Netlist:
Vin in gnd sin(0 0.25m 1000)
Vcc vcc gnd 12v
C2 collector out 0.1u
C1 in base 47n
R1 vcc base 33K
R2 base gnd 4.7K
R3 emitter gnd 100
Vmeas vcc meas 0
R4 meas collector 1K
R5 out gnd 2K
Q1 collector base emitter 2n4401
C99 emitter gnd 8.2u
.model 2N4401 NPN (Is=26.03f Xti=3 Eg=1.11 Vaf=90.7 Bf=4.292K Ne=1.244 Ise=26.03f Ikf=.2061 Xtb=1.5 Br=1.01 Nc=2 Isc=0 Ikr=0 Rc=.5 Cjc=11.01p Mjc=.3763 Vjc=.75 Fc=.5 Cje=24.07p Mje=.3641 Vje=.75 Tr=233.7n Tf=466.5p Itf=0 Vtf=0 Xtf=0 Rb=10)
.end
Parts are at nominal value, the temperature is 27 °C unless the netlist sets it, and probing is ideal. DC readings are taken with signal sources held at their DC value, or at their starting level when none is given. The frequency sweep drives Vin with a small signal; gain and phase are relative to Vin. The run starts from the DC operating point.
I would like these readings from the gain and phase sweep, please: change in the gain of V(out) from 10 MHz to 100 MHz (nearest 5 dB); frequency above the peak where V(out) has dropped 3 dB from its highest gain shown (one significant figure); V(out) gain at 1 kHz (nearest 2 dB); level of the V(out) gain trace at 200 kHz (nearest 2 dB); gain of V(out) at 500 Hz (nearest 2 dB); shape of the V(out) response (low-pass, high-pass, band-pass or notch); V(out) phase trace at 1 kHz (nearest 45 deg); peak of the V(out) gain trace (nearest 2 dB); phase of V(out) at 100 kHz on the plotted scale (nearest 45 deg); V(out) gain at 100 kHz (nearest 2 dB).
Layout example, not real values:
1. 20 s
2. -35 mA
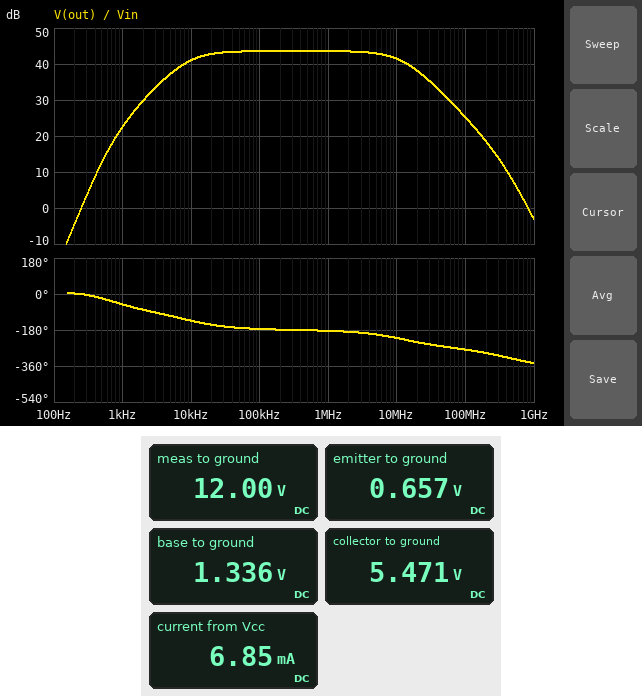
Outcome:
1. -15 dB
2. 10 MHz
3. 22 dB
4. 44 dB
5. 12 dB
6. band-pass
7. -45 deg
8. 44 dB
9. -180 deg
10. 44 dB
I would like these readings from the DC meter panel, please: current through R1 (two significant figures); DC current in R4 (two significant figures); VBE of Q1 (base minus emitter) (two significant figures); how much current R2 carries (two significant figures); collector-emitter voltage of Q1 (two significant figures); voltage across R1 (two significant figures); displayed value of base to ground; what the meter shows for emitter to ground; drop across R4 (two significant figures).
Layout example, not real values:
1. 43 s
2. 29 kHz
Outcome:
1. 320 µA
2. 6.5 mA
3. 680 mV
4. 280 µA
5. 4.8 V
6. 11 V
7. 1.336 V
8. 0.657 V
9. 6.5 V
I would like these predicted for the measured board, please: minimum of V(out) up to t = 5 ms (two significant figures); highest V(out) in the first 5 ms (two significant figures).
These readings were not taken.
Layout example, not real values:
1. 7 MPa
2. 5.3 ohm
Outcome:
1. -3.4 mV
2. 3.4 mV
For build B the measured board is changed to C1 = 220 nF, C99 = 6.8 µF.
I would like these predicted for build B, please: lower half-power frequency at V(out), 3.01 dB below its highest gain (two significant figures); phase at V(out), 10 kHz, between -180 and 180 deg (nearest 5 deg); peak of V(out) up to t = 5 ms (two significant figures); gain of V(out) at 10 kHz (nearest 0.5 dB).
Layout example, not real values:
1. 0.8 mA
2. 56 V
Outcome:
1. 6.6 kHz
2. -145 deg
3. 5.2 mV
4. 42.0 dB
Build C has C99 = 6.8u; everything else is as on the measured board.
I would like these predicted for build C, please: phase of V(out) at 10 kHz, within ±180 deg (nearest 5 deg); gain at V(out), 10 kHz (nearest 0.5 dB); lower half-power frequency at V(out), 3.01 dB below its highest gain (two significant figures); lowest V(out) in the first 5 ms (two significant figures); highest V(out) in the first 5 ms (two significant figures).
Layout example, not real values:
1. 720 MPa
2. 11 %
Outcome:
1. -130 deg
2. 40.5 dB
3. 9.9 kHz
4. -3.0 mV
5. 3.0 mV
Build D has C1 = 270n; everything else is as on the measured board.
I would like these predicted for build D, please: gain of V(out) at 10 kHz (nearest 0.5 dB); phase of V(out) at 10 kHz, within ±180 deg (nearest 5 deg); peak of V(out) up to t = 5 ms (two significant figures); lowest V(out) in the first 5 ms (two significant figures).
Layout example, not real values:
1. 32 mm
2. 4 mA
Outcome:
1. 42.5 dB
2. -150 deg
3. 6.2 mV
4. -6.3 mV
